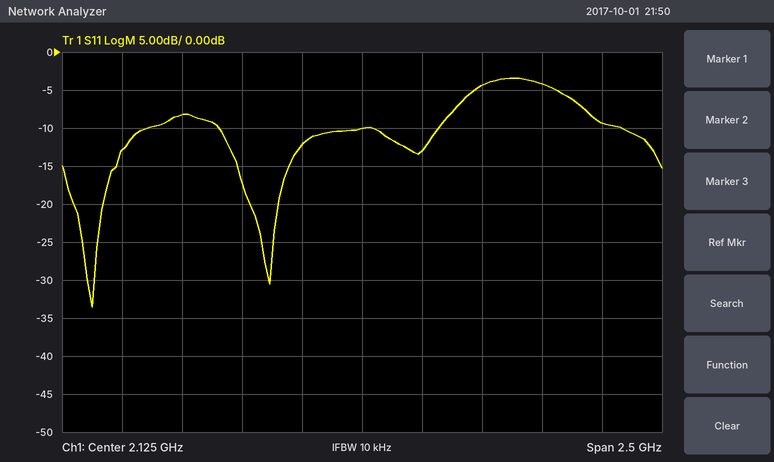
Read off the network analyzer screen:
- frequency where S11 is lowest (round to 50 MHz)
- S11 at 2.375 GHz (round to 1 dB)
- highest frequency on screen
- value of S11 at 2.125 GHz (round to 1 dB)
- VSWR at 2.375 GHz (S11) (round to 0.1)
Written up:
1.00 GHz
-13 dB
3.375 GHz
-10 dB
1.6
